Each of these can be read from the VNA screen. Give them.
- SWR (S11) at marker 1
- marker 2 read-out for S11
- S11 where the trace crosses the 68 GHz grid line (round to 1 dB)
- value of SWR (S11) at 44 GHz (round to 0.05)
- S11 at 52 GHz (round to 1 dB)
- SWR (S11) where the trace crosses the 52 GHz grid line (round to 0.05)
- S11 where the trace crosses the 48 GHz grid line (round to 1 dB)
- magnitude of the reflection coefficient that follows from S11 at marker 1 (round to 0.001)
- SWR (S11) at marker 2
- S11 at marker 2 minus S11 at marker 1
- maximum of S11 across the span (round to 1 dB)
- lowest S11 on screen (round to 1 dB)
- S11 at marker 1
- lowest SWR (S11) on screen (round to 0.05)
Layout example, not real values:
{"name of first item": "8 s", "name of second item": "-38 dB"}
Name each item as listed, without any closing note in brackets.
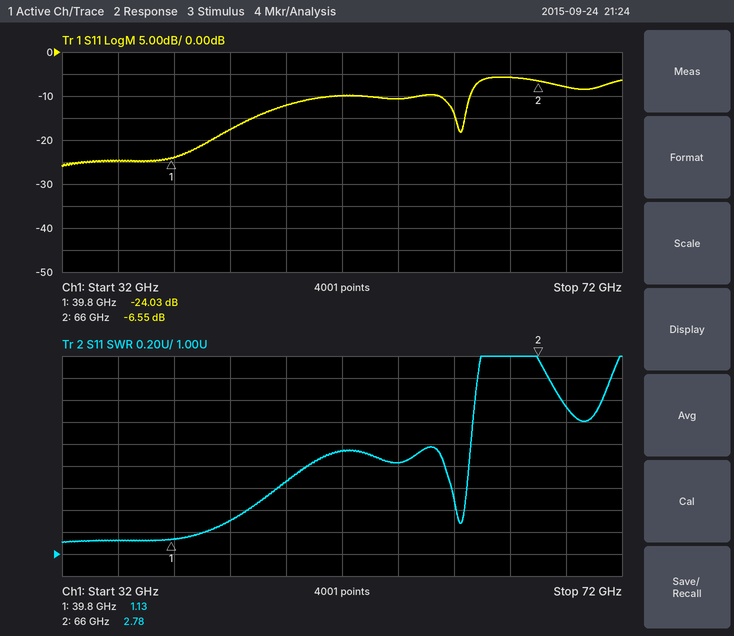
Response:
{"SWR (S11) at marker 1": "1.13", "marker 2 read-out for S11": "-6.55 dB", "S11 where the trace crosses the 68 GHz grid line": "-8 dB", "value of SWR (S11) at 44 GHz": "1.30", "S11 at 52 GHz": "-10 dB", "SWR (S11) where the trace crosses the 52 GHz grid line": "1.95", "S11 where the trace crosses the 48 GHz grid line": "-12 dB", "magnitude of the reflection coefficient that follows from S11 at marker 1": "0.063", "SWR (S11) at marker 2": "2.78", "S11 at marker 2 minus S11 at marker 1": "17.48 dB", "maximum of S11 across the span": "-6 dB", "lowest S11 on screen": "-26 dB", "S11 at marker 1": "-24.03 dB", "lowest SWR (S11) on screen": "1.10"}
